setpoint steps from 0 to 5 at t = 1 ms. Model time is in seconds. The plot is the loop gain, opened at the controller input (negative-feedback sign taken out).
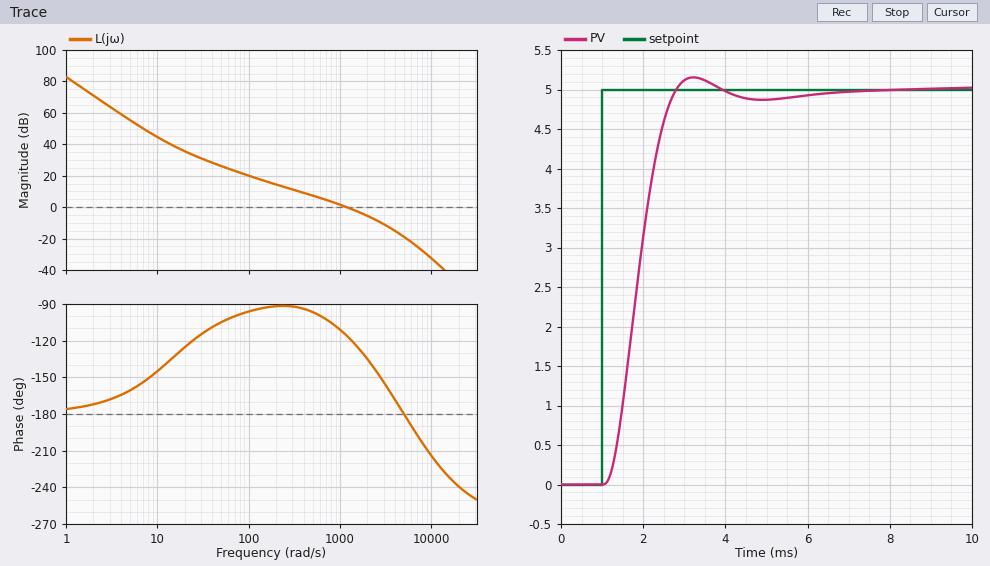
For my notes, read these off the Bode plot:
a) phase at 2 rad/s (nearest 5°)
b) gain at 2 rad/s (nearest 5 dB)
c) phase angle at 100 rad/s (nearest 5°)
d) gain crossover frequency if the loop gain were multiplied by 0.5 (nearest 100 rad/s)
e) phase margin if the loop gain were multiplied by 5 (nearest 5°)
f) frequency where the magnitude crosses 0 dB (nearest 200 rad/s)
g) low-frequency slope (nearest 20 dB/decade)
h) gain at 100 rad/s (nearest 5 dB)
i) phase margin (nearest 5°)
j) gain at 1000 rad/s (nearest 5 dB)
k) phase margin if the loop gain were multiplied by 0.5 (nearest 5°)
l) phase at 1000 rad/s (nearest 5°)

-170°
70 dB
-95°
600 rad/s
15°
1200 rad/s
-40 dB/decade
20 dB
65°
0 dB
80°
-110°
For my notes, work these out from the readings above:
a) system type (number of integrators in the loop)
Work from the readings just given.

2
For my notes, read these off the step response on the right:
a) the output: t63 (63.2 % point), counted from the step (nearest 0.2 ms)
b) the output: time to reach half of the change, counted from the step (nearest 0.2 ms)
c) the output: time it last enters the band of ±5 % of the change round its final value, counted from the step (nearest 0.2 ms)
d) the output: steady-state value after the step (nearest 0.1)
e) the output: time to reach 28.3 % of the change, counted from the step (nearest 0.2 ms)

1.0 ms
0.8 ms
1.6 ms
5.0
0.6 ms
